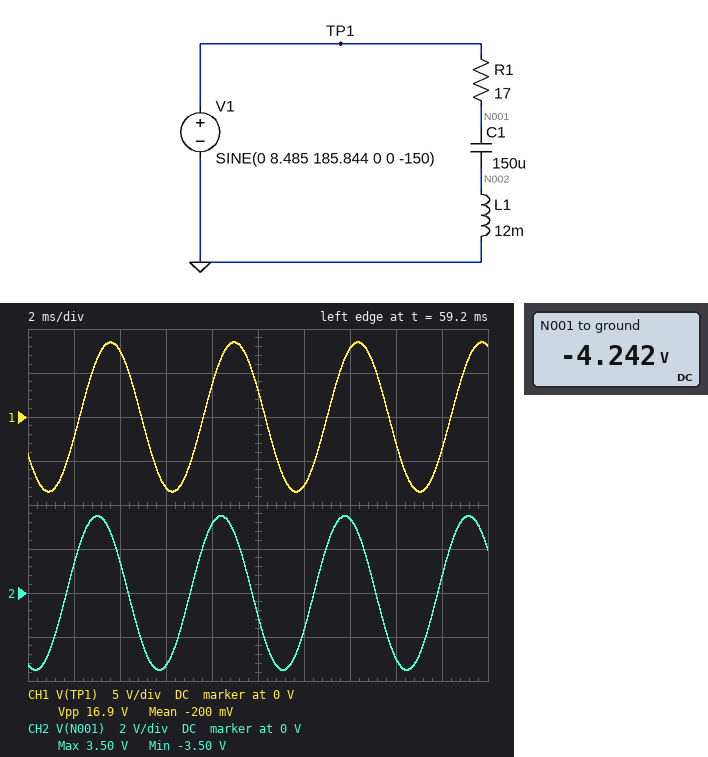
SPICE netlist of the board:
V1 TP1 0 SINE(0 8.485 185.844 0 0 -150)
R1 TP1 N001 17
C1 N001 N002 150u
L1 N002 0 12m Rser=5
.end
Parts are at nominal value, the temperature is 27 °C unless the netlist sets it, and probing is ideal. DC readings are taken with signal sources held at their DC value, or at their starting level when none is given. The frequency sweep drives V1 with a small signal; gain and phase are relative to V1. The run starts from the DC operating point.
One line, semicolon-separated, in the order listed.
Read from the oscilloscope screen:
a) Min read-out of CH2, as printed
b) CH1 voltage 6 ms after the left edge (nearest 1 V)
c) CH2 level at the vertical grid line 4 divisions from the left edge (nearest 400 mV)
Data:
-3.50 V; -8 V; 3.2 V
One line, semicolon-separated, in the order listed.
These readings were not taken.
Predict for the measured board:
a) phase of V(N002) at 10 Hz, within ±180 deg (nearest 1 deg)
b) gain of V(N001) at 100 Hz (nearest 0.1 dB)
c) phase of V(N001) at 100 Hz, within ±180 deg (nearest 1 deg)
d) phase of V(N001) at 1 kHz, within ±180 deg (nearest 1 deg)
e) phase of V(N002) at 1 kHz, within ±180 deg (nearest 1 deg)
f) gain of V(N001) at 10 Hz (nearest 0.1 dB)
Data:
87 deg; -11.6 dB; -24 deg; 13 deg; 13 deg; -0.2 dB
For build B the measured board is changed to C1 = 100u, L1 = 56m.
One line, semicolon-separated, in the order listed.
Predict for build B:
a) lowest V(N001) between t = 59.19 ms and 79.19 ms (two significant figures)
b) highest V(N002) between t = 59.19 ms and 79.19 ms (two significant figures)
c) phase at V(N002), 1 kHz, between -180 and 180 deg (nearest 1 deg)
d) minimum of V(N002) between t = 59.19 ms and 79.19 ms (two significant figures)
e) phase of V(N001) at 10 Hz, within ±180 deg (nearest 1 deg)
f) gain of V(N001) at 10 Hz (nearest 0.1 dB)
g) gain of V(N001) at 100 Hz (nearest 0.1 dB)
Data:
-7.9 V; 9.1 V; 3 deg; -9.1 V; -6 deg; -0.1 dB; -3.3 dB
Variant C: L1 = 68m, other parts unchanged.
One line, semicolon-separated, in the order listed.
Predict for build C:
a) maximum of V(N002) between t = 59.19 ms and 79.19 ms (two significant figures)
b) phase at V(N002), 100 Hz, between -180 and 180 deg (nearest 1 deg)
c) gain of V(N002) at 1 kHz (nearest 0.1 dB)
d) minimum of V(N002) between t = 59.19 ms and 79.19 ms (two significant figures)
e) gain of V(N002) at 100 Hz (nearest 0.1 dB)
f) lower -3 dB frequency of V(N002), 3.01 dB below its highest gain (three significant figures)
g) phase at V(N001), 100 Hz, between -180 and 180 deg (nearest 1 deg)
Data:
8.8 V; 28 deg; 0 dB; -8.8 V; 0.9 dB; 42.2 Hz; 26 deg
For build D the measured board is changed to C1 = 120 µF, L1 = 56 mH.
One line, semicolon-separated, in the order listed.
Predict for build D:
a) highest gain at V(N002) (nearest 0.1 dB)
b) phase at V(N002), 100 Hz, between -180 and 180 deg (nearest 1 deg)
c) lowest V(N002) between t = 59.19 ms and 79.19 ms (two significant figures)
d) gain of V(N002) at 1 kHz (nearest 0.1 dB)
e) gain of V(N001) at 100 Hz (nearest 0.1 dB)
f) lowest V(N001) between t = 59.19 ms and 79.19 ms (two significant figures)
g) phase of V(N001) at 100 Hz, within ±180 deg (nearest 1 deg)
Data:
1.3 dB; 37 deg; -8.9 V; 0 dB; -2.8 dB; -8.0 V; 32 deg
